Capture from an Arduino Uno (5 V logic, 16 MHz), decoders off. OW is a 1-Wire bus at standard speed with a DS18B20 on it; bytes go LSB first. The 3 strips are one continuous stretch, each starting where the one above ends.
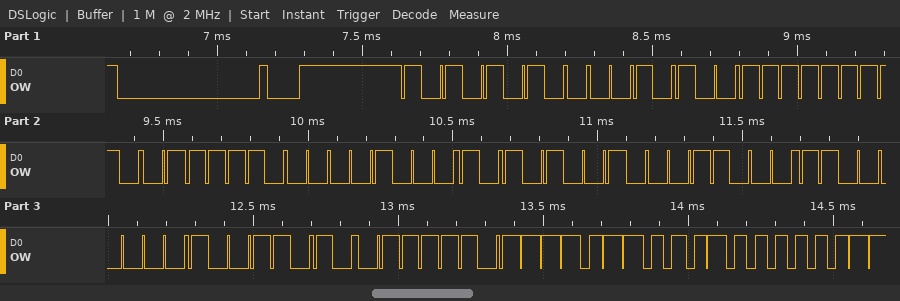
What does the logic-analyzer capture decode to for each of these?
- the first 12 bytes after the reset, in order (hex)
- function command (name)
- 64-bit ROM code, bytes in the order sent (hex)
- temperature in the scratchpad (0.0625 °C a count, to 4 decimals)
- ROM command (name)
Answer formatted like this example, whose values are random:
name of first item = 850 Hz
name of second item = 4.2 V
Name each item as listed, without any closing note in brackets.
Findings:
the first 12 bytes after the reset, in order = 55 28 FF 7C 10 95 18 03 59 BE 37 02
function command = Read Scratchpad
64-bit ROM code, bytes in the order sent = 28 FF 7C 10 95 18 03 59
temperature in the scratchpad = 35.4375 °C
ROM command = Match ROM
